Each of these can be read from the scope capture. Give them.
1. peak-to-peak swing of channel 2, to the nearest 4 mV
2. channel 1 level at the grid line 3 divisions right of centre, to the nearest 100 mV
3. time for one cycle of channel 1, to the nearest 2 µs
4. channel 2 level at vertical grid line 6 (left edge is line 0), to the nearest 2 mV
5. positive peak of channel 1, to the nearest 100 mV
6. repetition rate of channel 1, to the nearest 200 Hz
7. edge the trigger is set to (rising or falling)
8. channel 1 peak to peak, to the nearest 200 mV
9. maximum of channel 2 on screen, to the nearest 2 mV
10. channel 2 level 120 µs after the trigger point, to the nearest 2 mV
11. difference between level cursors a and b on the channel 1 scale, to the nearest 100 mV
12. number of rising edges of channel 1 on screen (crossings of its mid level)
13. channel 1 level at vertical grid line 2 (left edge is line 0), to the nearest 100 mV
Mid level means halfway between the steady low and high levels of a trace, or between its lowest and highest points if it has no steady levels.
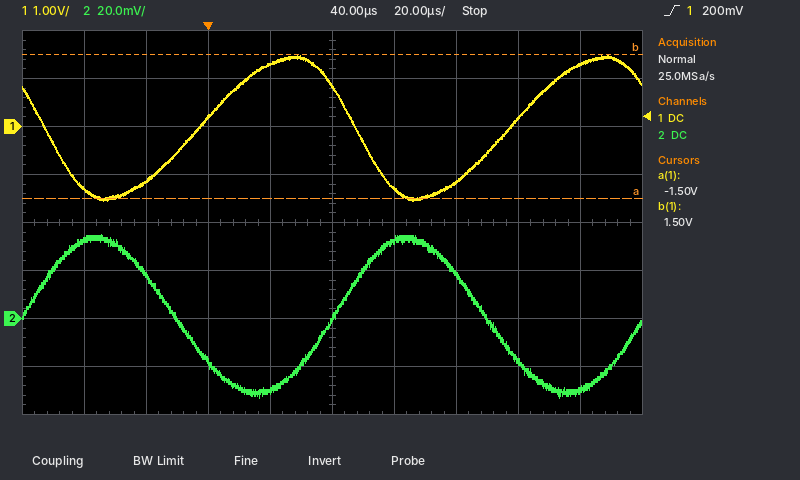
68 mV
200 mV
100 µs
32 mV
1.5 V
10.0 kHz
rising
3.0 V
36 mV
-30 mV
3.0 V
2
-1.1 V
